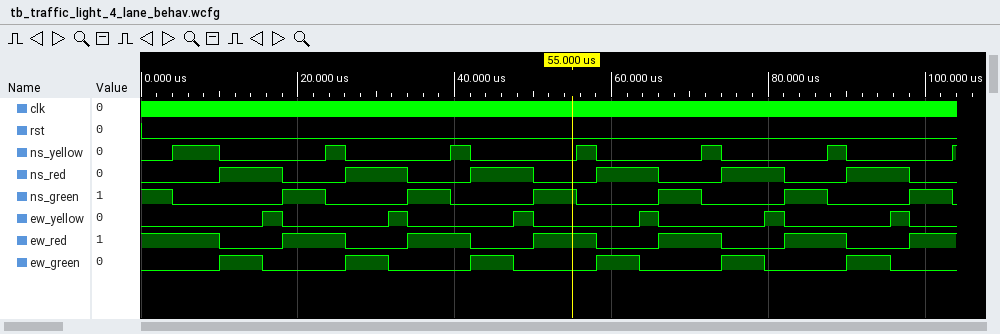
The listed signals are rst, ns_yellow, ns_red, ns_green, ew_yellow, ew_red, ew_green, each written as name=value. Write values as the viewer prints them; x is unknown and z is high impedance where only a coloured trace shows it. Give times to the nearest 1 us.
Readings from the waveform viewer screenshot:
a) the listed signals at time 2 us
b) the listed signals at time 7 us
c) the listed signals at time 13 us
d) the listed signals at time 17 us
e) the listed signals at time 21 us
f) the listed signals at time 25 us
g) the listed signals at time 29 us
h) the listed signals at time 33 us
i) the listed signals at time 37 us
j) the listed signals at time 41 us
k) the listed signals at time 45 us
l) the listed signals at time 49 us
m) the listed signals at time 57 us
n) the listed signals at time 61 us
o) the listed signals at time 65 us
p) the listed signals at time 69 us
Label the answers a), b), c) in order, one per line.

a) rst=0, ns_yellow=0, ns_red=0, ns_green=1, ew_yellow=0, ew_red=1, ew_green=0
b) rst=0, ns_yellow=1, ns_red=0, ns_green=0, ew_yellow=0, ew_red=1, ew_green=0
c) rst=0, ns_yellow=0, ns_red=1, ns_green=0, ew_yellow=0, ew_red=0, ew_green=1
d) rst=0, ns_yellow=0, ns_red=1, ns_green=0, ew_yellow=1, ew_red=0, ew_green=0
e) rst=0, ns_yellow=0, ns_red=0, ns_green=1, ew_yellow=0, ew_red=1, ew_green=0
f) rst=0, ns_yellow=1, ns_red=0, ns_green=0, ew_yellow=0, ew_red=1, ew_green=0
g) rst=0, ns_yellow=0, ns_red=1, ns_green=0, ew_yellow=0, ew_red=0, ew_green=1
h) rst=0, ns_yellow=0, ns_red=1, ns_green=0, ew_yellow=1, ew_red=0, ew_green=0
i) rst=0, ns_yellow=0, ns_red=0, ns_green=1, ew_yellow=0, ew_red=1, ew_green=0
j) rst=0, ns_yellow=1, ns_red=0, ns_green=0, ew_yellow=0, ew_red=1, ew_green=0
k) rst=0, ns_yellow=0, ns_red=1, ns_green=0, ew_yellow=0, ew_red=0, ew_green=1
l) rst=0, ns_yellow=0, ns_red=1, ns_green=0, ew_yellow=1, ew_red=0, ew_green=0
m) rst=0, ns_yellow=1, ns_red=0, ns_green=0, ew_yellow=0, ew_red=1, ew_green=0
n) rst=0, ns_yellow=0, ns_red=1, ns_green=0, ew_yellow=0, ew_red=0, ew_green=1
o) rst=0, ns_yellow=0, ns_red=1, ns_green=0, ew_yellow=1, ew_red=0, ew_green=0
p) rst=0, ns_yellow=0, ns_red=0, ns_green=1, ew_yellow=0, ew_red=1, ew_green=0
